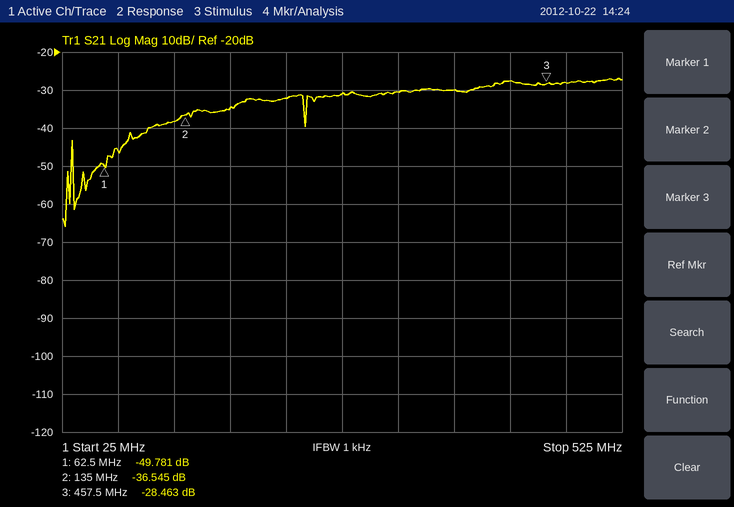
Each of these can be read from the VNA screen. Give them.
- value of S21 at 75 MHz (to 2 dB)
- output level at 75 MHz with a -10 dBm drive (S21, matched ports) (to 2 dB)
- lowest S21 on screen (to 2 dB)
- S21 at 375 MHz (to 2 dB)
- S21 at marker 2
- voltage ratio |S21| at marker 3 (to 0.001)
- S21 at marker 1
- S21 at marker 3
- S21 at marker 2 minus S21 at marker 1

-46 dB
-56 dBm
-66 dB
-30 dB
-36.545 dB
0.038
-49.781 dB
-28.463 dB
13.236 dB
